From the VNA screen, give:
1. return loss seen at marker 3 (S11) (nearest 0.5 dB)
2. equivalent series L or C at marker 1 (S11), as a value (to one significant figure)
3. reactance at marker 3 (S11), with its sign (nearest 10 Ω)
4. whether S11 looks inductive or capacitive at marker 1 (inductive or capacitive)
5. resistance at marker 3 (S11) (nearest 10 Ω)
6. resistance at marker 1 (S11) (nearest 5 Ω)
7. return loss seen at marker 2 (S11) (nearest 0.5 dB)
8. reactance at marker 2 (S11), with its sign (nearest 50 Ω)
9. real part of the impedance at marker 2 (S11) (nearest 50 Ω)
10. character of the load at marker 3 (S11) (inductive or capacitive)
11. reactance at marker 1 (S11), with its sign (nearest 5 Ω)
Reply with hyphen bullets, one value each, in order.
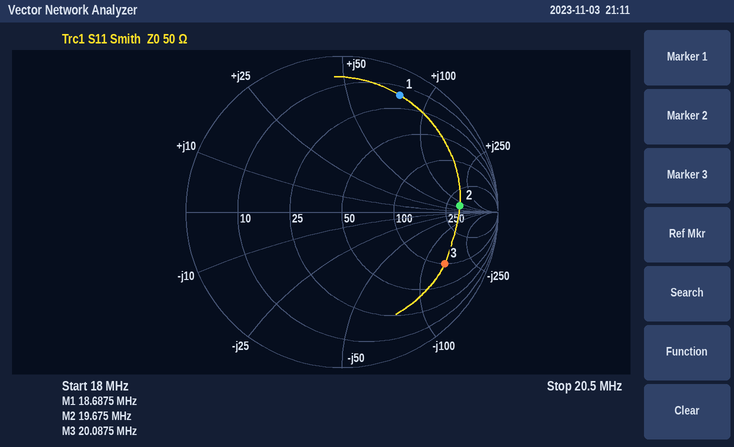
- 2.5 dB
- 700 nH
- -150 Ω
- inductive
- 100 Ω
- 15 Ω
- 2.5 dB
- +50 Ω
- 350 Ω
- capacitive
- +80 Ω
